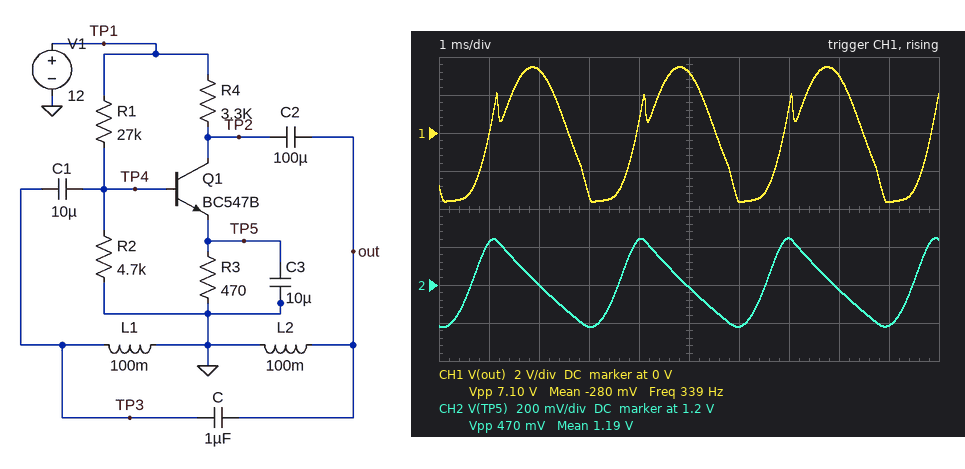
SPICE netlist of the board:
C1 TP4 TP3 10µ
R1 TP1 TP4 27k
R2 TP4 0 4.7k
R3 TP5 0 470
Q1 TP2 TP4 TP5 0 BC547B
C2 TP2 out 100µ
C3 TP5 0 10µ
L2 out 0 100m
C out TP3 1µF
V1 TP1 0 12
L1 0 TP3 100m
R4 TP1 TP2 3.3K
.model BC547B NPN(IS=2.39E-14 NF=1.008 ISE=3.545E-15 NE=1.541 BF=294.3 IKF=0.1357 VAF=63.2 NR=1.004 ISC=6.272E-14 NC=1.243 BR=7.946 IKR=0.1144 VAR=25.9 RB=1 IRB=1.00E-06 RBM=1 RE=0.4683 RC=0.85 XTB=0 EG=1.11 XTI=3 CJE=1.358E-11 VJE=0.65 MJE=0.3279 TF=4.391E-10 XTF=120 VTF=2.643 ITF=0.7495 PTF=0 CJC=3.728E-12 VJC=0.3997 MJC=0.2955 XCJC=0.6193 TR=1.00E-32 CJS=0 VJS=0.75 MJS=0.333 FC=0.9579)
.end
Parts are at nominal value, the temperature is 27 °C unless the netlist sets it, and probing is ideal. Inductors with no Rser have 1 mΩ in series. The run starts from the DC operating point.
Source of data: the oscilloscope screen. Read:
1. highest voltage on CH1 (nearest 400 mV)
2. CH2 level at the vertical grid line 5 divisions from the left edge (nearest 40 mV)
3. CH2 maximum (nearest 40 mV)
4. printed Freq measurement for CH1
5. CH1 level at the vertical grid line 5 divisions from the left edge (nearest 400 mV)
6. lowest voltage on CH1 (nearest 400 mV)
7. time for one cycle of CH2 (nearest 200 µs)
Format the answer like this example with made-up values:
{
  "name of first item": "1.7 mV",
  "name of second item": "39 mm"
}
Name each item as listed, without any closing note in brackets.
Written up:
{
  "highest voltage on CH1": "3.6 V",
  "CH2 level at the vertical grid line 5 divisions from the left edge": "1.20 V",
  "CH2 maximum": "1.44 V",
  "printed Freq measurement for CH1": "339 Hz",
  "CH1 level at the vertical grid line 5 divisions from the left edge": "3.2 V",
  "lowest voltage on CH1": "-3.6 V",
  "time for one cycle of CH2": "3.0 ms"
}
